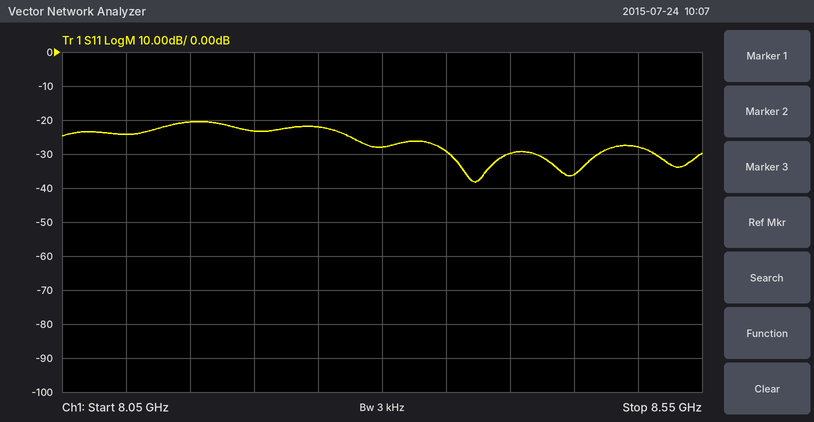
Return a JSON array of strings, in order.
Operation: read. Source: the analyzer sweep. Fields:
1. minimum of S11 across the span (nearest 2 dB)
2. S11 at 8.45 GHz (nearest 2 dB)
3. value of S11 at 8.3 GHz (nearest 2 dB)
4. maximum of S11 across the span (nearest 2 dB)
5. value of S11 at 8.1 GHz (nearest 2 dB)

["-38 dB", "-36 dB", "-28 dB", "-20 dB", "-24 dB"]
